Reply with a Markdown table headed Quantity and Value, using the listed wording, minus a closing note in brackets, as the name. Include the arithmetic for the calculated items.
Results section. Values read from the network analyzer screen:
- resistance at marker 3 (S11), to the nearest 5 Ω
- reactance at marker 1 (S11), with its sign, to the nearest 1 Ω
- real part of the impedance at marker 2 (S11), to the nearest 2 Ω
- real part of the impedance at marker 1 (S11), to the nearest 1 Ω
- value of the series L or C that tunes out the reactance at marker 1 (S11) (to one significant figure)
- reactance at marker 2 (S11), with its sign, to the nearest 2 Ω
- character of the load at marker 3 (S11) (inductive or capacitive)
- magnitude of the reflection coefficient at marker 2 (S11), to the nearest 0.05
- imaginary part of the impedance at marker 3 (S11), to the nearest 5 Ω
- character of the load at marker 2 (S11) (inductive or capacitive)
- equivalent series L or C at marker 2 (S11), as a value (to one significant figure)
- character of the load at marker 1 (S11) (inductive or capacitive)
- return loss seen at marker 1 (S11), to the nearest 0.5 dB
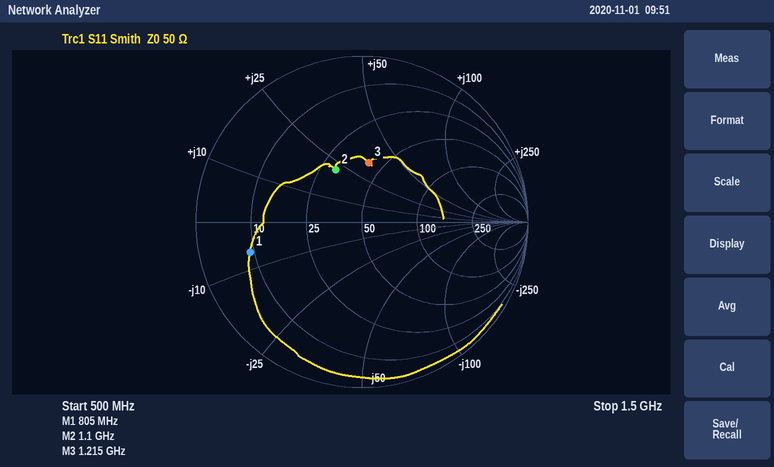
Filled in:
| Quantity | Value |
|---|---|
| resistance at marker 3 (S11), to the nearest 5 Ω | 40 Ω |
| reactance at marker 1 (S11), with its sign, to the nearest 1 Ω | -6 Ω |
| real part of the impedance at marker 2 (S11), to the nearest 2 Ω | 30 Ω |
| real part of the impedance at marker 1 (S11), to the nearest 1 Ω | 9 Ω |
| value of the series L or C that tunes out the reactance at marker 1 (S11) | L = 6 Ω/(2π × 805 MHz) ≈ 1 nH |
| reactance at marker 2 (S11), with its sign, to the nearest 2 Ω | +22 Ω |
| character of the load at marker 3 (S11) | inductive |
| magnitude of the reflection coefficient at marker 2 (S11), to the nearest 0.05 | 0.35 |
| imaginary part of the impedance at marker 3 (S11), to the nearest 5 Ω | +35 Ω |
| character of the load at marker 2 (S11) | inductive |
| equivalent series L or C at marker 2 (S11), as a value | L = 22 Ω/(2π × 1.1 GHz) ≈ 3 nH |
| character of the load at marker 1 (S11) | capacitive |
| return loss seen at marker 1 (S11), to the nearest 0.5 dB | 3.0 dB |
